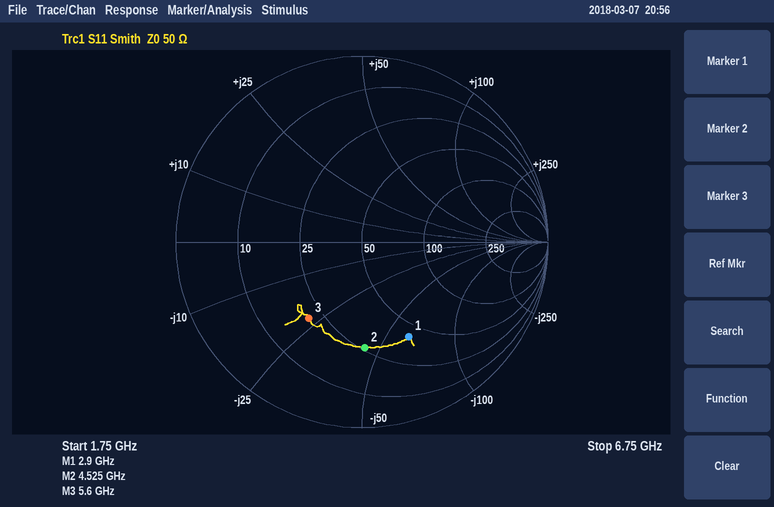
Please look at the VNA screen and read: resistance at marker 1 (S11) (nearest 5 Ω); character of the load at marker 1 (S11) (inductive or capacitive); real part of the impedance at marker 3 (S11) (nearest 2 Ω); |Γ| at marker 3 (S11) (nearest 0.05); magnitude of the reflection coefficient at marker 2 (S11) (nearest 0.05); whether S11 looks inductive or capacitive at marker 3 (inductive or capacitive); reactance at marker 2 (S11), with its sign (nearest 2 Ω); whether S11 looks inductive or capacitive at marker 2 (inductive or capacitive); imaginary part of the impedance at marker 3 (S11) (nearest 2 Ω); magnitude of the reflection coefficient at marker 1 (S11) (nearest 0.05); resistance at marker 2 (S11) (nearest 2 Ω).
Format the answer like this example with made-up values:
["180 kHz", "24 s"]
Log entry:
["40 Ω", "capacitive", "20 Ω", "0.50", "0.55", "capacitive", "-44 Ω", "capacitive", "-22 Ω", "0.55", "26 Ω"]
